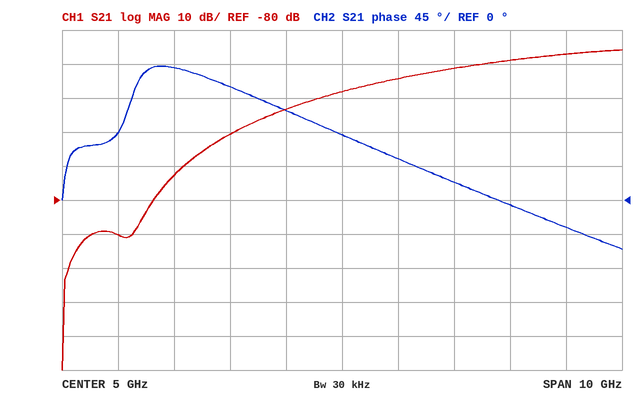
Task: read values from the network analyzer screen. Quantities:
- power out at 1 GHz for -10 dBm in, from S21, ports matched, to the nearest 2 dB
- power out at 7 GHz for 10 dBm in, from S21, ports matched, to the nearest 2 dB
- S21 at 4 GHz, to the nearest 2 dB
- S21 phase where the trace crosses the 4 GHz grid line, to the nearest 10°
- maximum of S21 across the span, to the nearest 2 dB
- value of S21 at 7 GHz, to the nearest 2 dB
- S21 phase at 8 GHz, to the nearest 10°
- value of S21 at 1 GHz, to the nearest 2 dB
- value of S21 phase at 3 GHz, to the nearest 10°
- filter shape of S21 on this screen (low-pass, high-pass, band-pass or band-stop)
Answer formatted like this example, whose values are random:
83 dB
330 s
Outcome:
-100 dBm
-32 dBm
-54 dB
120°
-36 dB
-42 dB
-10°
-90 dB
150°
high-pass
